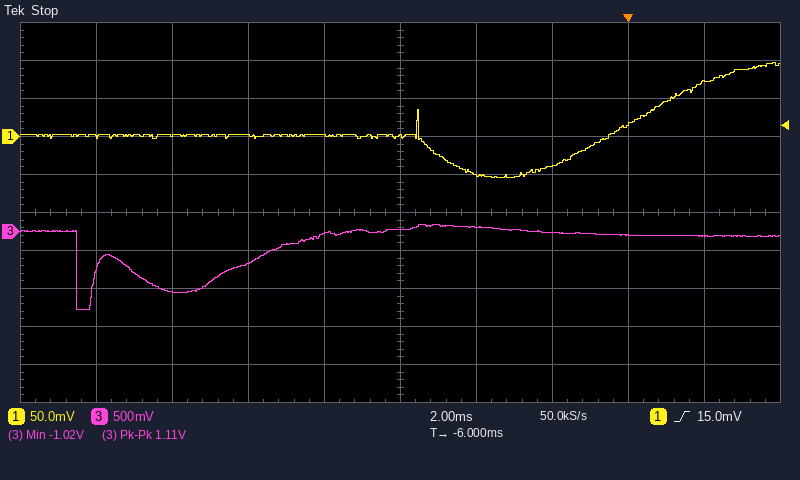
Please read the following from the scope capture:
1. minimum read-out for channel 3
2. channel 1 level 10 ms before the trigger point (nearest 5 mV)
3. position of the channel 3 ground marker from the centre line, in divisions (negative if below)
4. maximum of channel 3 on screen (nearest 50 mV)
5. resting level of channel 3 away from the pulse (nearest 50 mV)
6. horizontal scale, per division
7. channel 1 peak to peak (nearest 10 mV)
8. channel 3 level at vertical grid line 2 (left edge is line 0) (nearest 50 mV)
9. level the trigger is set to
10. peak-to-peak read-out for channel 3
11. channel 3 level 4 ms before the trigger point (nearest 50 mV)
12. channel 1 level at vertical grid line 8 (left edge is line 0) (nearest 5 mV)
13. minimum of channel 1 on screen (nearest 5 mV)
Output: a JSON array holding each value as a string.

["-1.02 V", "0 mV", "-0.5 div", "100 mV", "-50 mV", "2 ms", "150 mV", "-800 mV", "15.0 mV", "1.11 V", "50 mV", "15 mV", "-55 mV"]
